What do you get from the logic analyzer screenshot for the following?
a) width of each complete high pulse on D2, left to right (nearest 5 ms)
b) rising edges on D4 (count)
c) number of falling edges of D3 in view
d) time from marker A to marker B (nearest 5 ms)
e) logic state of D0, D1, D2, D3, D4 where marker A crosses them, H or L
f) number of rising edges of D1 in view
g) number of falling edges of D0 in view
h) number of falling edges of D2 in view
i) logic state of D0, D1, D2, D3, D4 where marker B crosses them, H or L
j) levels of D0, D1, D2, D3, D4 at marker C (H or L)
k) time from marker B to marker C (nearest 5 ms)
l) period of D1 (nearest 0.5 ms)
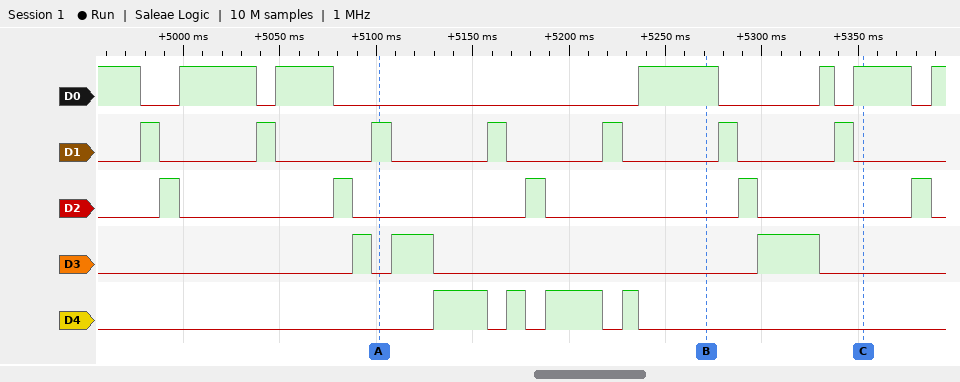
10 ms, 10 ms, 10 ms, 10 ms, 10 ms
4
3
170 ms
D0=L, D1=H, D2=L, D3=L, D4=L
7
6
5
D0=H, D1=L, D2=L, D3=L, D4=L
D0=H, D1=L, D2=L, D3=L, D4=L
80 ms
60 ms
